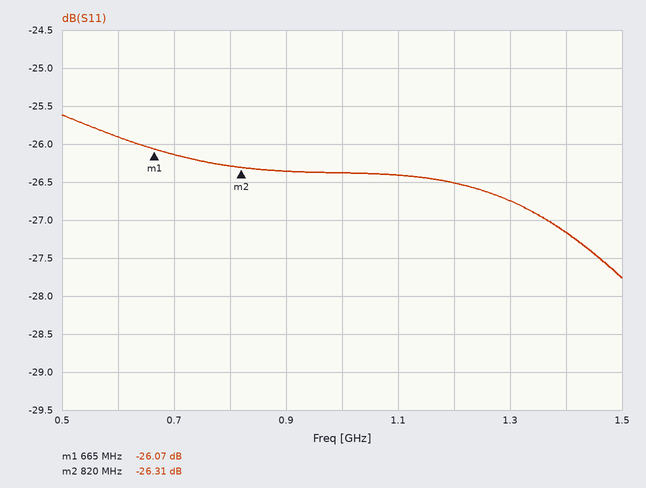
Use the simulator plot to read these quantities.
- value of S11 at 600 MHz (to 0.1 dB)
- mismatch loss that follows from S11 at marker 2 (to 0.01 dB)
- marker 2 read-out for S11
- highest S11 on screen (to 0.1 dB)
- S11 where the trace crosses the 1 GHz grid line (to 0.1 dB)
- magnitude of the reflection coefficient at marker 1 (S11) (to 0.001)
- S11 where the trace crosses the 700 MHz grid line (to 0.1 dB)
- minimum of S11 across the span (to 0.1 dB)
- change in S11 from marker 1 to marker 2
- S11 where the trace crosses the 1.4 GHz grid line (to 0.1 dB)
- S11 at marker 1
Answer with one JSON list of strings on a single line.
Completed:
["-25.9 dB", "0.01 dB", "-26.31 dB", "-25.6 dB", "-26.4 dB", "0.050", "-26.1 dB", "-27.8 dB", "-0.24 dB", "-27.2 dB", "-26.07 dB"]
